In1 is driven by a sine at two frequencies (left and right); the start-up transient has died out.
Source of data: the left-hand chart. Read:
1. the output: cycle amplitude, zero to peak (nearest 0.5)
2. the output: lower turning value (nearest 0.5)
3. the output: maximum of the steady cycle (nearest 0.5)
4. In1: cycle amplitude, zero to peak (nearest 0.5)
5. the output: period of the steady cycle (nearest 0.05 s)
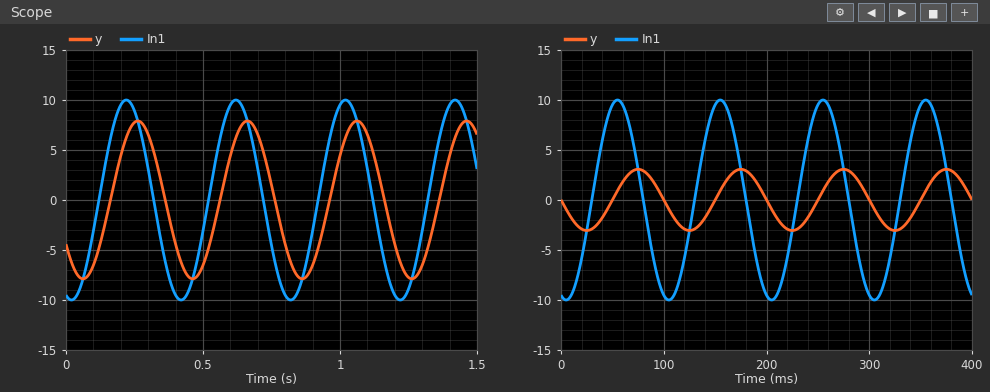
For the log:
8.0
-8.0
8.0
10.0
0.40 s
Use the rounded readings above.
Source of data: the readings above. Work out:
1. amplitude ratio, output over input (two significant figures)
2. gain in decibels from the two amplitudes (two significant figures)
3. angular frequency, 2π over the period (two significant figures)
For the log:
0.80
-1.9 dB
16 rad/s
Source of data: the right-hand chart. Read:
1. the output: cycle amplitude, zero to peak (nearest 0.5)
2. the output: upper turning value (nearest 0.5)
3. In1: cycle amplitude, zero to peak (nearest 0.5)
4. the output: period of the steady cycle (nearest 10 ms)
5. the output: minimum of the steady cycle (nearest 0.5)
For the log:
3.0
3.0
10.0
100 ms
-3.0
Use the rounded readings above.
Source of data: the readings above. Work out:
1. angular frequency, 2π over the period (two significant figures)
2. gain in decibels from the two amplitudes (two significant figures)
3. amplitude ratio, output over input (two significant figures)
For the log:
0.063 rad/ms
-10 dB
0.30
